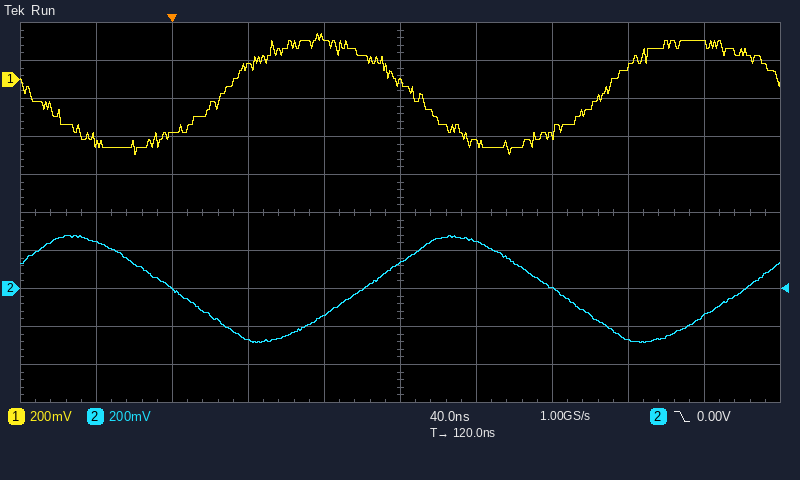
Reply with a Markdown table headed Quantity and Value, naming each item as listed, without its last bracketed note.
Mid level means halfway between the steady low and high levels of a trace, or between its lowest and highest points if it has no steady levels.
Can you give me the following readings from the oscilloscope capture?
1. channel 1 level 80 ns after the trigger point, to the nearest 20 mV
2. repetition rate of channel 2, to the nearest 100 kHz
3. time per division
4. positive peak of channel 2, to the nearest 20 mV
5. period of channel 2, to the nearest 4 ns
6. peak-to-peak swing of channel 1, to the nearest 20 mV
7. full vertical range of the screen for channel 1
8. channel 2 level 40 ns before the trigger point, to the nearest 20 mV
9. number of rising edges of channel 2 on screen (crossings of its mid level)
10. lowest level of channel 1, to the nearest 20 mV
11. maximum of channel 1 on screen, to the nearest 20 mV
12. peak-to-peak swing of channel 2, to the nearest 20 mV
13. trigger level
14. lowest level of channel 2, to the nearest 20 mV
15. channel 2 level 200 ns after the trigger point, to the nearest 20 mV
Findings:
| Quantity | Value |
|---|---|
| channel 1 level 80 ns after the trigger point, to the nearest 20 mV | 220 mV |
| repetition rate of channel 2, to the nearest 100 kHz | 5.0 MHz |
| time per division | 40 ns |
| positive peak of channel 2, to the nearest 20 mV | 280 mV |
| period of channel 2, to the nearest 4 ns | 200 ns |
| peak-to-peak swing of channel 1, to the nearest 20 mV | 640 mV |
| full vertical range of the screen for channel 1 | 2 V |
| channel 2 level 40 ns before the trigger point, to the nearest 20 mV | 240 mV |
| number of rising edges of channel 2 on screen | 2 |
| lowest level of channel 1, to the nearest 20 mV | -400 mV |
| maximum of channel 1 on screen, to the nearest 20 mV | 240 mV |
| peak-to-peak swing of channel 2, to the nearest 20 mV | 560 mV |
| trigger level | 0.00 V |
| lowest level of channel 2, to the nearest 20 mV | -280 mV |
| channel 2 level 200 ns after the trigger point, to the nearest 20 mV | 0 mV |
